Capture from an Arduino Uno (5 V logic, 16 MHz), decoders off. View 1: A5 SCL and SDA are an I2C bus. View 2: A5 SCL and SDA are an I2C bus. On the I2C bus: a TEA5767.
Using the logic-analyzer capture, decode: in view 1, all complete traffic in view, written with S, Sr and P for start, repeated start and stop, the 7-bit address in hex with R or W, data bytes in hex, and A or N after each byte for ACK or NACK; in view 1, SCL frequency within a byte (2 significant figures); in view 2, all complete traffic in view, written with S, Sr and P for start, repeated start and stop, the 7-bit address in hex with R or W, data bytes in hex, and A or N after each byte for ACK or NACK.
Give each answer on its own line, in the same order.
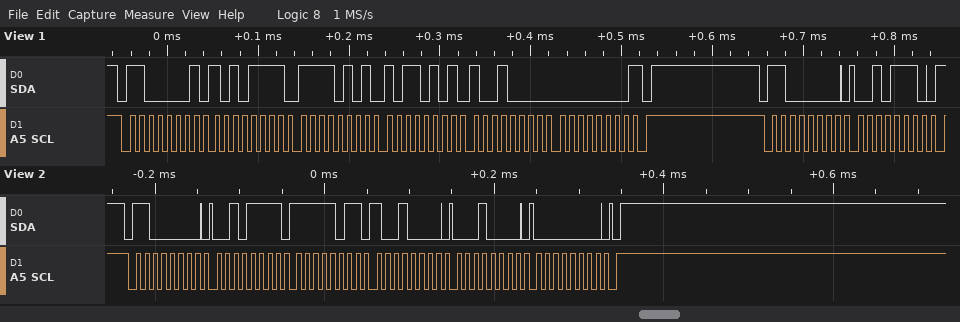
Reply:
S 60R A AF A F5 A B5 A 90 A 00 N P S 60W A 2E A
100 kHz
S 60W A 2F A FB A 90 A 10 A 00 A P
